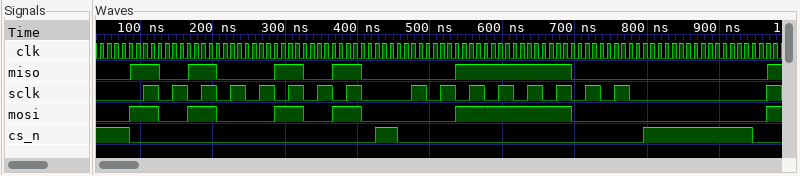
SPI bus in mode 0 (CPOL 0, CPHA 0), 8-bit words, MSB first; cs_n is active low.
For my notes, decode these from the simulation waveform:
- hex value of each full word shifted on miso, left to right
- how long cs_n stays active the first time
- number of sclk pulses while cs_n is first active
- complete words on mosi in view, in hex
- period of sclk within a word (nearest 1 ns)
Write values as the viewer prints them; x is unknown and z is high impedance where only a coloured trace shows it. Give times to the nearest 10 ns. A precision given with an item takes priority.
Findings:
A5, 3C
340 ns
8
A5, 3C
40 ns
